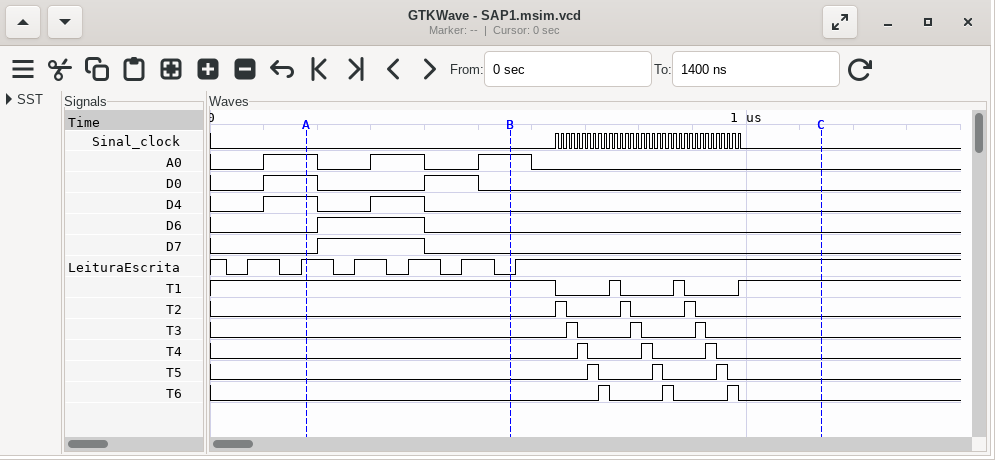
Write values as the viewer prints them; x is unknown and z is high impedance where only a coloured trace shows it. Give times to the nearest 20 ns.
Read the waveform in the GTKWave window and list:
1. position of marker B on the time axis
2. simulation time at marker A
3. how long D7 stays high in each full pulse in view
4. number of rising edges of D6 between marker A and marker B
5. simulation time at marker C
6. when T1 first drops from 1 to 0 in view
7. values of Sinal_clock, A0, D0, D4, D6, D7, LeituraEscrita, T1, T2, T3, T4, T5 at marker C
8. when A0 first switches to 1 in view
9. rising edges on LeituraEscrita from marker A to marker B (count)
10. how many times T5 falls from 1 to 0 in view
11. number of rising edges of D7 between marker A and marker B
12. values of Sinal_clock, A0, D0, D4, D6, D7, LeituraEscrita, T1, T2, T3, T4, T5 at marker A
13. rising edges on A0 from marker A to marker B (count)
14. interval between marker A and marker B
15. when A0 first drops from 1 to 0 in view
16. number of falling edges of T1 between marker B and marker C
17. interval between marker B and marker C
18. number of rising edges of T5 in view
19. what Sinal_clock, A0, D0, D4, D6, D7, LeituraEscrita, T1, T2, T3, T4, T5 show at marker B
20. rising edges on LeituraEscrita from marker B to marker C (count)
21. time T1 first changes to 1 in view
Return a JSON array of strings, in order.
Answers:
["560 ns", "180 ns", "200 ns", "1", "1140 ns", "640 ns", "Sinal_clock=0, A0=0, D0=0, D4=0, D6=0, D7=0, LeituraEscrita=1, T1=1, T2=0, T3=0, T4=0, T5=0", "100 ns", "3", "3", "1", "Sinal_clock=0, A0=1, D0=1, D4=1, D6=0, D7=0, LeituraEscrita=1, T1=1, T2=0, T3=0, T4=0, T5=0", "2", "380 ns", "200 ns", "3", "580 ns", "3", "Sinal_clock=0, A0=1, D0=0, D4=0, D6=0, D7=0, LeituraEscrita=0, T1=1, T2=0, T3=0, T4=0, T5=0", "1", "740 ns"]
